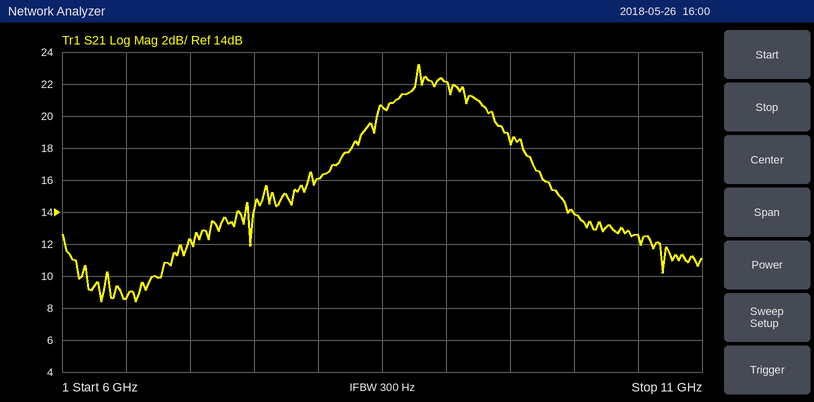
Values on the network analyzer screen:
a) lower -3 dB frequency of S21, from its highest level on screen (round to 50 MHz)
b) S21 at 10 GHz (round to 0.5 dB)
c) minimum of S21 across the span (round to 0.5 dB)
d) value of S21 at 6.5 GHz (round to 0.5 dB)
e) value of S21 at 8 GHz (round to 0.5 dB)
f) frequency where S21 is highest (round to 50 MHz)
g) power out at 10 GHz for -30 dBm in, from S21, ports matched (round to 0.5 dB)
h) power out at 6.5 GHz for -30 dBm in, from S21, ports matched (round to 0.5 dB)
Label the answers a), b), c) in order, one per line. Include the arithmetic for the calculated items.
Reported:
a) 8.45 GHz
b) 14.0 dB
c) 8.5 dB
d) 8.5 dB
e) 16.0 dB
f) 8.80 GHz
g) -30 dBm + (14.0 dB) = -16.0 dBm
h) -30 dBm + (8.5 dB) = -21.5 dBm
